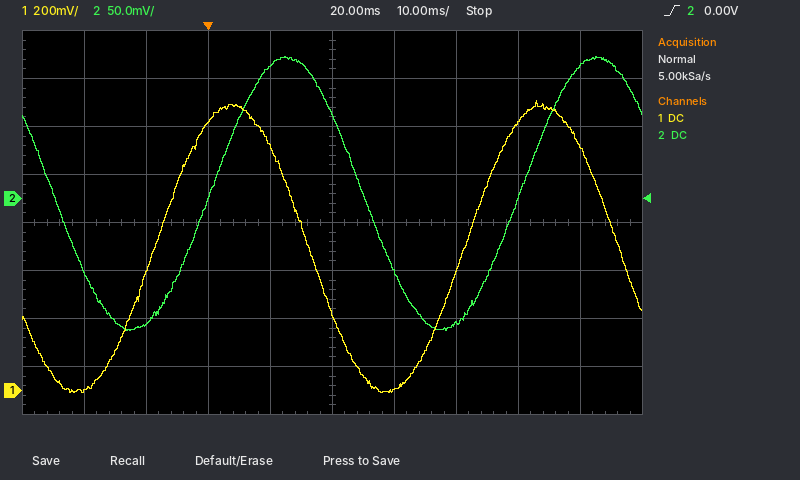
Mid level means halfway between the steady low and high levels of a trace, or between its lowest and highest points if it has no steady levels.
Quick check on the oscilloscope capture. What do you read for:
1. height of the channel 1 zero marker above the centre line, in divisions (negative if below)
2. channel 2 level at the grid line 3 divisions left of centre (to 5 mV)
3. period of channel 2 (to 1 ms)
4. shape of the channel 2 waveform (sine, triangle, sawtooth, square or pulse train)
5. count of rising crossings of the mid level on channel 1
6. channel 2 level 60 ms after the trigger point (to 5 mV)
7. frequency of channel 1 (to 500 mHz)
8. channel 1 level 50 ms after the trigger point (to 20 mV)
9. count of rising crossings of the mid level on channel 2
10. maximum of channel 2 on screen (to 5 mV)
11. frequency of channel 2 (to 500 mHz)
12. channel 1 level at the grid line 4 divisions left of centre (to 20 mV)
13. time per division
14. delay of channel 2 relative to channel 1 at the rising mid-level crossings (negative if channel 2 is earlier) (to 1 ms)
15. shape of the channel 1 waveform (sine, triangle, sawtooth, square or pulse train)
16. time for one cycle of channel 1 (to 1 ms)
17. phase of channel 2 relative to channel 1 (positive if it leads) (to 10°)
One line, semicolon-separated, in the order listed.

-3.5 div; -130 mV; 50 ms; sine; 2; 140 mV; 20.0 Hz; 1.12 V; 2; 150 mV; 20.0 Hz; 0 mV; 10 ms; +9 ms; sine; 50 ms; -60°
